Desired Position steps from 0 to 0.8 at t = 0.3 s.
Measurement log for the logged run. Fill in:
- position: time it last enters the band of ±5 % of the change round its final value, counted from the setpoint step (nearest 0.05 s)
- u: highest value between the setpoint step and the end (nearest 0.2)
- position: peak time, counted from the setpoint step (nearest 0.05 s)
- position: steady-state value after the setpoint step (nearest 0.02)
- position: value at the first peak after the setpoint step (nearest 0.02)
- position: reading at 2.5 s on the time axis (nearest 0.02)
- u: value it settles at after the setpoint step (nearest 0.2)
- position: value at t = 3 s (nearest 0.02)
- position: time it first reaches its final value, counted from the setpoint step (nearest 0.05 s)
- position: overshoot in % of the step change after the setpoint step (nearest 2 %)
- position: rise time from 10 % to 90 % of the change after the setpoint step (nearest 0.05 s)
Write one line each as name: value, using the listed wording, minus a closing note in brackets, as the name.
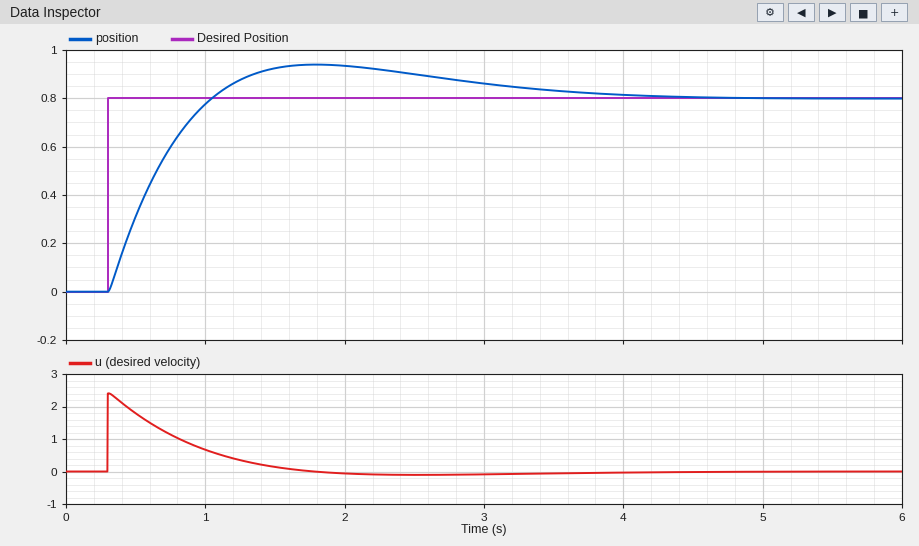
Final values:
position: time it last enters the band of ±5 % of the change round its final value, counted from the setpoint step: 3.05 s
u: highest value between the setpoint step and the end: 2.4
position: peak time, counted from the setpoint step: 1.50 s
position: steady-state value after the setpoint step: 0.80
position: value at the first peak after the setpoint step: 0.94
position: reading at 2.5 s on the time axis: 0.90
u: value it settles at after the setpoint step: 0.0
position: value at t = 3 s: 0.86
position: time it first reaches its final value, counted from the setpoint step: 0.75 s
position: overshoot in % of the step change after the setpoint step: 18 %
position: rise time from 10 % to 90 % of the change after the setpoint step: 0.55 s
